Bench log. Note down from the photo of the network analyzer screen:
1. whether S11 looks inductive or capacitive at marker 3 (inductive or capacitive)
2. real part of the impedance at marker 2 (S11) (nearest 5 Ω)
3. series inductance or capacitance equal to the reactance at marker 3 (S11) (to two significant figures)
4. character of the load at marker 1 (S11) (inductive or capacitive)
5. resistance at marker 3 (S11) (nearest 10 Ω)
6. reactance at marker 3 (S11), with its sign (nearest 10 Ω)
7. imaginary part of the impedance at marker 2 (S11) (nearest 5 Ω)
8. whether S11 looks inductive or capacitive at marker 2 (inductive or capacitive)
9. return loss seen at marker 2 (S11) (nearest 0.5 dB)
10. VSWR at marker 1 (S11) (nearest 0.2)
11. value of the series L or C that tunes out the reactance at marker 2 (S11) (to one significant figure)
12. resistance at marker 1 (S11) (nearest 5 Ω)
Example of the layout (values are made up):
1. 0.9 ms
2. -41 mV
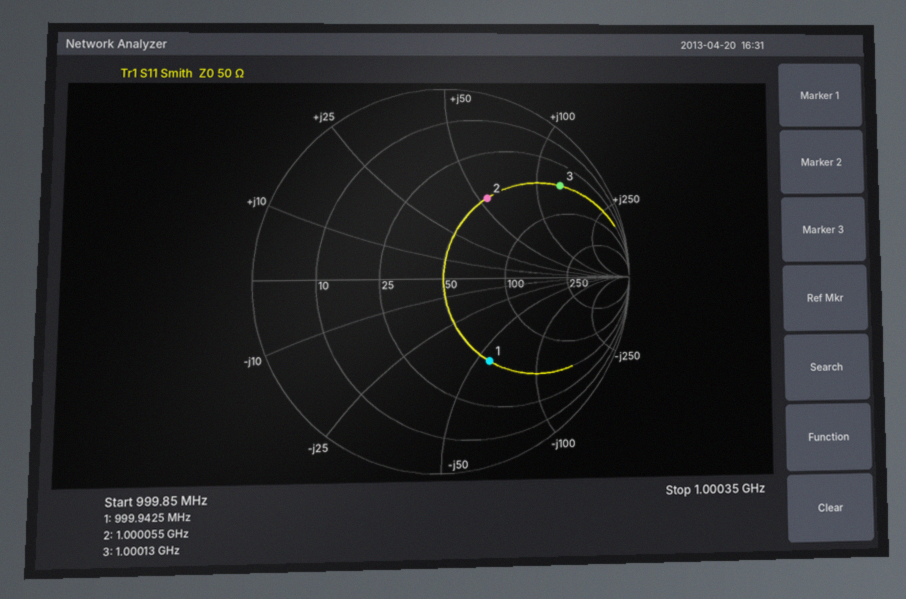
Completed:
1. inductive
2. 50 Ω
3. 21 nH
4. capacitive
5. 50 Ω
6. +130 Ω
7. +55 Ω
8. inductive
9. 6.5 dB
10. 3.0
11. 3 pF
12. 50 Ω
